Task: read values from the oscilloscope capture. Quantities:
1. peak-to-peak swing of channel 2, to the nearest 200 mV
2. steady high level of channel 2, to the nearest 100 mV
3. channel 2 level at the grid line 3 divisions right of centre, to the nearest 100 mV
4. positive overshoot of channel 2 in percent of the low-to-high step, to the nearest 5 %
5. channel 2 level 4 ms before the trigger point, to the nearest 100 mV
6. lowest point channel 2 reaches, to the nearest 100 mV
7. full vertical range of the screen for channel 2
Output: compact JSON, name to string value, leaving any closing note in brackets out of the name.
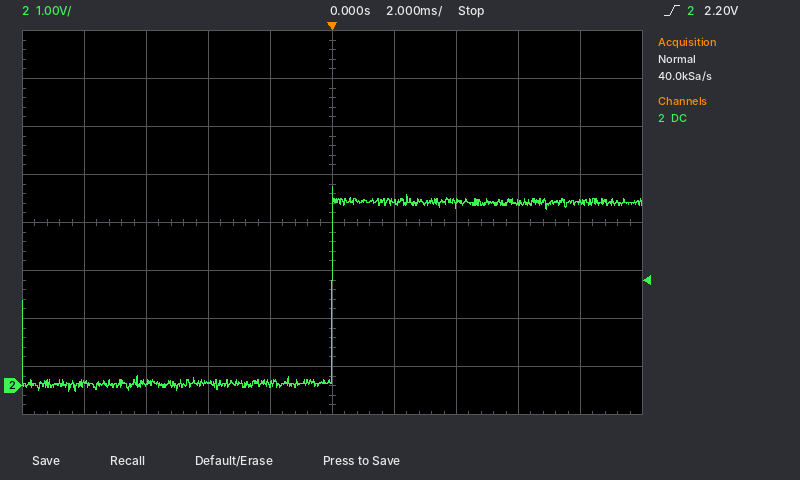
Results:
{"peak-to-peak swing of channel 2, to the nearest 200 mV": "4.2 V", "steady high level of channel 2, to the nearest 100 mV": "3.8 V", "channel 2 level at the grid line 3 divisions right of centre, to the nearest 100 mV": "3.8 V", "positive overshoot of channel 2 in percent of the low-to-high step, to the nearest 5 %": "10 %", "channel 2 level 4 ms before the trigger point, to the nearest 100 mV": "100 mV", "lowest point channel 2 reaches, to the nearest 100 mV": "-100 mV", "full vertical range of the screen for channel 2": "8 V"}
